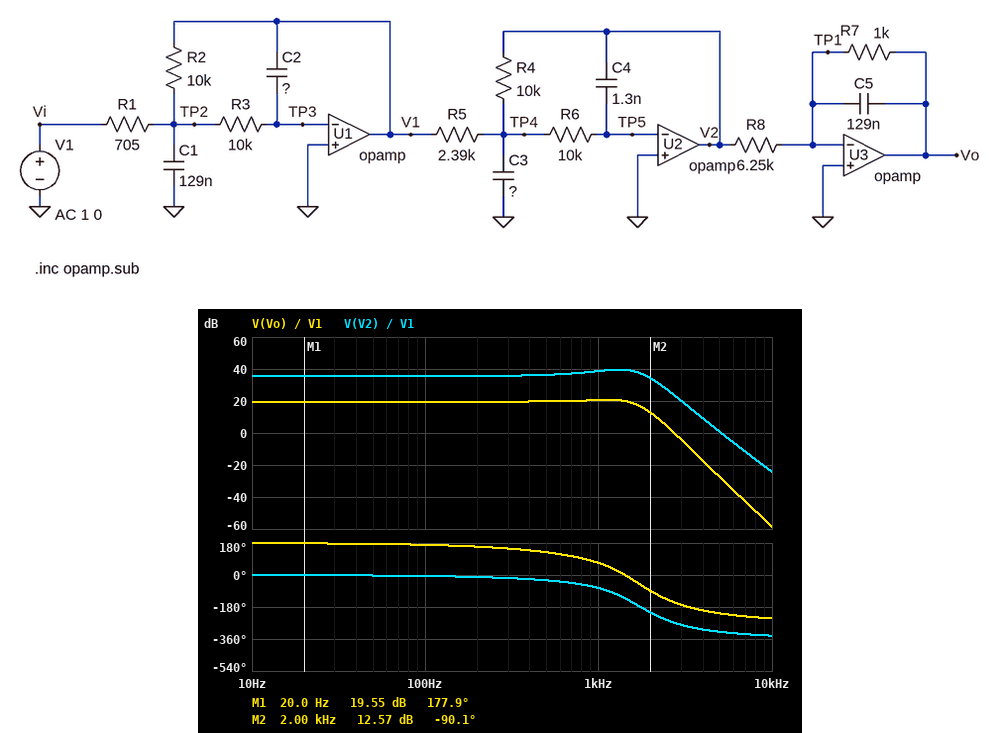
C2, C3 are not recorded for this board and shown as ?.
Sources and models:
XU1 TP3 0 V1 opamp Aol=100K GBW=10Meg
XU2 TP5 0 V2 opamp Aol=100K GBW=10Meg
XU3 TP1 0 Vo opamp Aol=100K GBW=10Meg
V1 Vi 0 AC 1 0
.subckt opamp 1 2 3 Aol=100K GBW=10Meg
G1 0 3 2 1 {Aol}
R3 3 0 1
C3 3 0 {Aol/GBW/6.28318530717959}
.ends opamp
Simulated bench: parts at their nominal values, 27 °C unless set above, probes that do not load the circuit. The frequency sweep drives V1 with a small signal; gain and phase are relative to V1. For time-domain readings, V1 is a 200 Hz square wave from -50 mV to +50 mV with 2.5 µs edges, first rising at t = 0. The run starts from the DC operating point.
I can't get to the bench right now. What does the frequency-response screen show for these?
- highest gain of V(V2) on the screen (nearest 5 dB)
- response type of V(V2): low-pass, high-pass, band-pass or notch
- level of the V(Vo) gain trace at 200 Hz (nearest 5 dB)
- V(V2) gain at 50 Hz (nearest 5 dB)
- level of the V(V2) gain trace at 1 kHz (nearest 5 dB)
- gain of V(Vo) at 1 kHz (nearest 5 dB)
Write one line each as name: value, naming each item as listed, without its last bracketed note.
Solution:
highest gain of V(V2) on the screen: 40 dB
response type of V(V2): low-pass, high-pass, band-pass or notch: low-pass
level of the V(Vo) gain trace at 200 Hz: 20 dB
V(V2) gain at 50 Hz: 35 dB
level of the V(V2) gain trace at 1 kHz: 40 dB
gain of V(Vo) at 1 kHz: 20 dB
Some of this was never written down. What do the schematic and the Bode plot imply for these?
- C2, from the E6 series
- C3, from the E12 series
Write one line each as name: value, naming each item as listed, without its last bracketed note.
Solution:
C2, from the E6 series: 470 pF
C3, from the E12 series: 82 nF
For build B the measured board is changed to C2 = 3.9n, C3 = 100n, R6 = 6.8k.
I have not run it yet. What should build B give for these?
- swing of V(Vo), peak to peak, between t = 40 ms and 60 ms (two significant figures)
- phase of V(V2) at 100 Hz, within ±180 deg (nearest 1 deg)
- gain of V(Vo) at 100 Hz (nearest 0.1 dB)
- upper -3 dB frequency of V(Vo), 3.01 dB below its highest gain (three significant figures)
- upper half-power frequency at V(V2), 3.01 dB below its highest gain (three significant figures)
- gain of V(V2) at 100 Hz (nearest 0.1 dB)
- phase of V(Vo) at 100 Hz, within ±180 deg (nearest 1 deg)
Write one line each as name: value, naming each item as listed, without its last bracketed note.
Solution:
swing of V(Vo), peak to peak, between t = 40 ms and 60 ms: 920 mV
phase of V(V2) at 100 Hz, within ±180 deg: -24 deg
gain of V(Vo) at 100 Hz: 19.1 dB
upper -3 dB frequency of V(Vo), 3.01 dB below its highest gain: 286 Hz
upper half-power frequency at V(V2), 3.01 dB below its highest gain: 302 Hz
gain of V(V2) at 100 Hz: 35.0 dB
phase of V(Vo) at 100 Hz, within ±180 deg: 151 deg
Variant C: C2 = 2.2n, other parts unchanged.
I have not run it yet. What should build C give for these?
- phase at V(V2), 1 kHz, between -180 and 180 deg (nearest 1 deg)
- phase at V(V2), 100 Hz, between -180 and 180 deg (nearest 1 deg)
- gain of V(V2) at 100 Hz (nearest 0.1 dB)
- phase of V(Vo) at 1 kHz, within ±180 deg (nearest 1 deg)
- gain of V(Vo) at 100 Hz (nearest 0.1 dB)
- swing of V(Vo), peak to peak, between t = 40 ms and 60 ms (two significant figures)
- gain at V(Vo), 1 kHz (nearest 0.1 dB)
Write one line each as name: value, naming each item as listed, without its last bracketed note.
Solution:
phase at V(V2), 1 kHz, between -180 and 180 deg: -134 deg
phase at V(V2), 100 Hz, between -180 and 180 deg: -16 deg
gain of V(V2) at 100 Hz: 35.4 dB
phase of V(Vo) at 1 kHz, within ±180 deg: 7 deg
gain of V(Vo) at 100 Hz: 19.4 dB
swing of V(Vo), peak to peak, between t = 40 ms and 60 ms: 950 mV
gain at V(Vo), 1 kHz: 12.6 dB
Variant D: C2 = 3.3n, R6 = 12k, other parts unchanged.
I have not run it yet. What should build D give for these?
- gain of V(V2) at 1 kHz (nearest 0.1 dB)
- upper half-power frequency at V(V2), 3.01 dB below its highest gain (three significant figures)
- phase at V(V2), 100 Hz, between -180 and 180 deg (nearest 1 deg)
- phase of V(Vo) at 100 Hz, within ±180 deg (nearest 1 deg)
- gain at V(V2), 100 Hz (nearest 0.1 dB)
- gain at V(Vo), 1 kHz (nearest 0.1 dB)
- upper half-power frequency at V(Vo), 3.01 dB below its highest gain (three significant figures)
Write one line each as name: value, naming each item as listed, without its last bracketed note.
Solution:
gain of V(V2) at 1 kHz: 27.0 dB
upper half-power frequency at V(V2), 3.01 dB below its highest gain: 380 Hz
phase at V(V2), 100 Hz, between -180 and 180 deg: -22 deg
phase of V(Vo) at 100 Hz, within ±180 deg: 153 deg
gain at V(V2), 100 Hz: 35.2 dB
gain at V(Vo), 1 kHz: 8.9 dB
upper half-power frequency at V(Vo), 3.01 dB below its highest gain: 349 Hz
